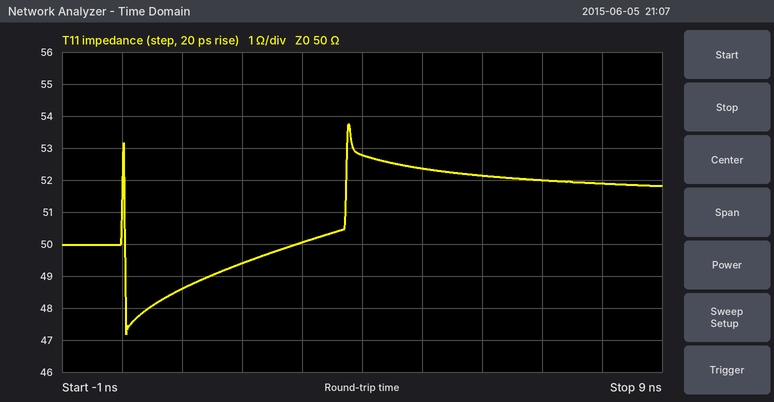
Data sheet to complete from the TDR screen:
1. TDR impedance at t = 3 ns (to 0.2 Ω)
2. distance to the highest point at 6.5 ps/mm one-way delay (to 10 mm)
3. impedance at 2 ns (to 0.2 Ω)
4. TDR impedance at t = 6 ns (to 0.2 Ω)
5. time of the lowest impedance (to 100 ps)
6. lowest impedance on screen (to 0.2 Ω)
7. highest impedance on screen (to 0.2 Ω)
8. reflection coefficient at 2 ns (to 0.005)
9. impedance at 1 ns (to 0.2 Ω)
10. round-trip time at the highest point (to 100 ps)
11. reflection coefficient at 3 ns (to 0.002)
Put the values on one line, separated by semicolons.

50.0 Ω; 290 mm; 49.4 Ω; 52.2 Ω; 100 ps; 47.2 Ω; 53.8 Ω; -0.005; 48.6 Ω; 3.8 ns; 0.000
